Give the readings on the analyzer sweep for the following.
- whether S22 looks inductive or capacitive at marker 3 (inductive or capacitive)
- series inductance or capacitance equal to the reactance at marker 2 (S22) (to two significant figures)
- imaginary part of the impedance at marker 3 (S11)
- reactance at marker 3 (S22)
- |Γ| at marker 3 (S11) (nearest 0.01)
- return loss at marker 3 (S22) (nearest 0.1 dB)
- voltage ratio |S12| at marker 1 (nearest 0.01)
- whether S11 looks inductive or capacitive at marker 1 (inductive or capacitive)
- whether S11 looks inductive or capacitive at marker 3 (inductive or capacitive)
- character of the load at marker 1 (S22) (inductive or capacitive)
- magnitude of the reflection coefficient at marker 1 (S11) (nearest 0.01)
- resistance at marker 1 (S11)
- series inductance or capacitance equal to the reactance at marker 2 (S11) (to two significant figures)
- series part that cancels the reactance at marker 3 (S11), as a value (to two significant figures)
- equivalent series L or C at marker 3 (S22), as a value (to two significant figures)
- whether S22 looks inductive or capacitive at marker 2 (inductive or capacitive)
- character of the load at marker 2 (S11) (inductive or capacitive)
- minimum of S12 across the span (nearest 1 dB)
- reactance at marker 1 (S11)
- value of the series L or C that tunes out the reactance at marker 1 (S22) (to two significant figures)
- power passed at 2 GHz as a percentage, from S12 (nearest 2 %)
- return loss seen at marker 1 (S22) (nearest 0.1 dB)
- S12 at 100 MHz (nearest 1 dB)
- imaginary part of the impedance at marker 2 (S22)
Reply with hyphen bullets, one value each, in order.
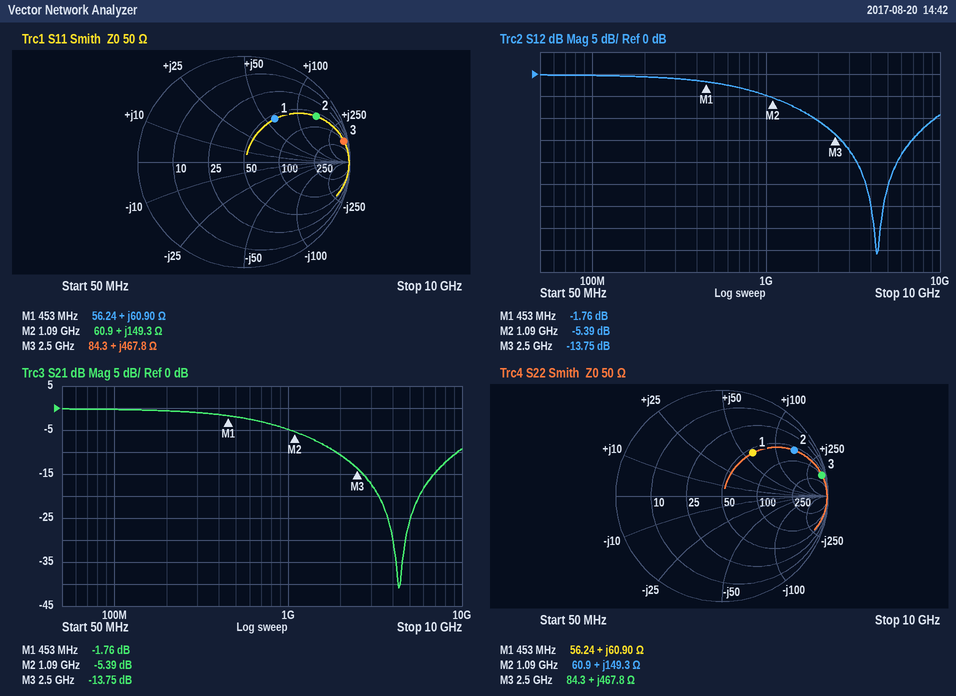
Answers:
- inductive
- 22 nH
- +467.8 Ω
- +467.8 Ω
- 0.96
- 0.3 dB
- 0.82
- inductive
- inductive
- inductive
- 0.50
- 56.24 Ω
- 22 nH
- 140 fF
- 30 nH
- inductive
- inductive
- -41 dB
- +60.90 Ω
- 5.8 pF
- 8 %
- 6.0 dB
- 0 dB
- +149.3 Ω
